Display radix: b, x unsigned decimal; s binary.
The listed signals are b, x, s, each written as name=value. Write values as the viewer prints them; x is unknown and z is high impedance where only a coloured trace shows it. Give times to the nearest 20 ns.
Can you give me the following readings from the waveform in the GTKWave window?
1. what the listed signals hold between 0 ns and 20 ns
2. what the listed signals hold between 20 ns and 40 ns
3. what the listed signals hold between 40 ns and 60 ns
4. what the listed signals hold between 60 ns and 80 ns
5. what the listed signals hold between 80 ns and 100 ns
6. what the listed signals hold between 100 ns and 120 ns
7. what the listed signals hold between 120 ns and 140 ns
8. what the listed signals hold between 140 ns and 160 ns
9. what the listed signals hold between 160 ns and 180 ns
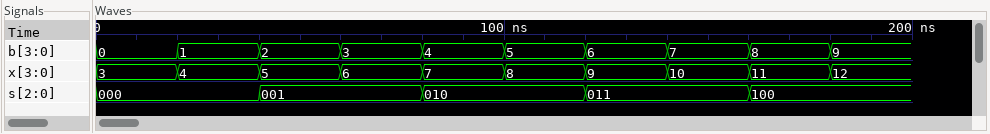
b=0, x=3, s=000
b=1, x=4, s=000
b=2, x=5, s=001
b=3, x=6, s=001
b=4, x=7, s=010
b=5, x=8, s=010
b=6, x=9, s=011
b=7, x=10, s=011
b=8, x=11, s=100
